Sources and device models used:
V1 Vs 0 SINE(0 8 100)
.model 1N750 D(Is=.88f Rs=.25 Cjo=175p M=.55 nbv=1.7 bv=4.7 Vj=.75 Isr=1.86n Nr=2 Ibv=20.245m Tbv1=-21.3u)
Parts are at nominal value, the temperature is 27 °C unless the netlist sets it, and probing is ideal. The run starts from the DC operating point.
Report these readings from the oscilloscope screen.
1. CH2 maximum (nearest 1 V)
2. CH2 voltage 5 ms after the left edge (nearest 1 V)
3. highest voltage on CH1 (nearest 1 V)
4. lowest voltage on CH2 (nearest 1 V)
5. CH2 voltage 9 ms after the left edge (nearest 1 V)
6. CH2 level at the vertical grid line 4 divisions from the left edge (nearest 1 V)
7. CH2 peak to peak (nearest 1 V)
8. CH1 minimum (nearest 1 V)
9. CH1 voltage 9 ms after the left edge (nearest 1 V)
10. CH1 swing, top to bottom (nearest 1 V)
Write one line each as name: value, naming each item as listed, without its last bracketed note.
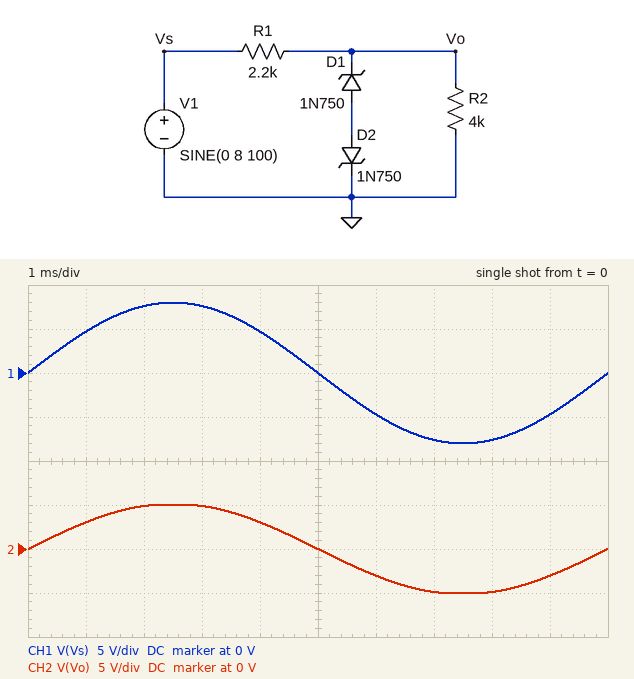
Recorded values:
CH2 maximum: 5 V
CH2 voltage 5 ms after the left edge: 0 V
highest voltage on CH1: 8 V
lowest voltage on CH2: -5 V
CH2 voltage 9 ms after the left edge: -3 V
CH2 level at the vertical grid line 4 divisions from the left edge: 3 V
CH2 peak to peak: 10 V
CH1 minimum: -8 V
CH1 voltage 9 ms after the left edge: -5 V
CH1 swing, top to bottom: 16 V
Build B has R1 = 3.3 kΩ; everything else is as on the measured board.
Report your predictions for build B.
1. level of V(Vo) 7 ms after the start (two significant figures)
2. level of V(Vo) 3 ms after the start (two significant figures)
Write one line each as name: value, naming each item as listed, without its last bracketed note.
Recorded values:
level of V(Vo) 7 ms after the start: -4.2 V
level of V(Vo) 3 ms after the start: 4.2 V
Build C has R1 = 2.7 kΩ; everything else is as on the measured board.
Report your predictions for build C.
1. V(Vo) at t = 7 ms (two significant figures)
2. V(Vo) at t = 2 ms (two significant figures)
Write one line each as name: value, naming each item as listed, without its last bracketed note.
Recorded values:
V(Vo) at t = 7 ms: -4.5 V
V(Vo) at t = 2 ms: 4.5 V
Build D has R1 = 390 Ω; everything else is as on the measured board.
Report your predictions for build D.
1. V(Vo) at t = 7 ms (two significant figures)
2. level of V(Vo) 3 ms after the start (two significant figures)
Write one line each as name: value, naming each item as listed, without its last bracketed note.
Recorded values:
V(Vo) at t = 7 ms: -5.4 V
level of V(Vo) 3 ms after the start: 5.4 V
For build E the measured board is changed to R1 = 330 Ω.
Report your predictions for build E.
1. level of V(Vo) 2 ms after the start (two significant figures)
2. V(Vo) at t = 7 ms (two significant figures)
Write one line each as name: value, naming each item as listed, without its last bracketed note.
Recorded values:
level of V(Vo) 2 ms after the start: 5.4 V
V(Vo) at t = 7 ms: -5.4 V
